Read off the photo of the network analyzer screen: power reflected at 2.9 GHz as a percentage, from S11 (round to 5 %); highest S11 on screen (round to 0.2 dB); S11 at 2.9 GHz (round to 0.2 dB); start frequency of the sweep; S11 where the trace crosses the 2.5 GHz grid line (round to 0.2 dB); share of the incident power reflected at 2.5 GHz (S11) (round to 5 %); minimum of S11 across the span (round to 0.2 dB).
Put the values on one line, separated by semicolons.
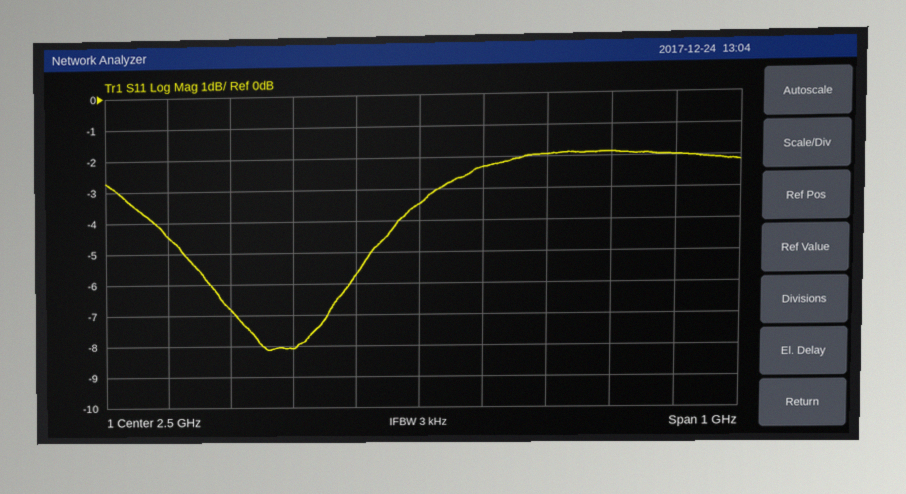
65 %; -1.8 dB; -2.0 dB; 2 GHz; -3.4 dB; 45 %; -8.2 dB
